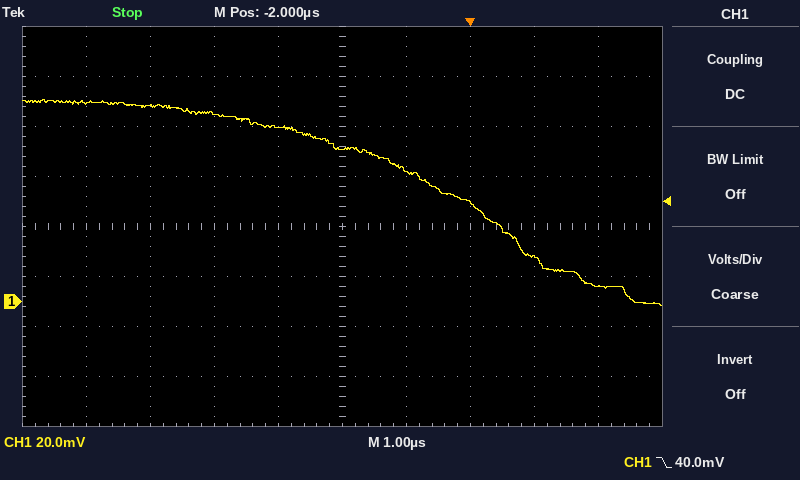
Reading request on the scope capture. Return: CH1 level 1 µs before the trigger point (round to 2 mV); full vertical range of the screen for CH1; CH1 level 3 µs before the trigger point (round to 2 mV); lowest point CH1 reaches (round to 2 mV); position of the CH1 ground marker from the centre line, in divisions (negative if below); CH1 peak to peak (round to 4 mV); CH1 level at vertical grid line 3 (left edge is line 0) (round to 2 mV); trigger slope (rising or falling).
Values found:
52 mV
160 mV
70 mV
-2 mV
-1.5 div
84 mV
76 mV
falling
